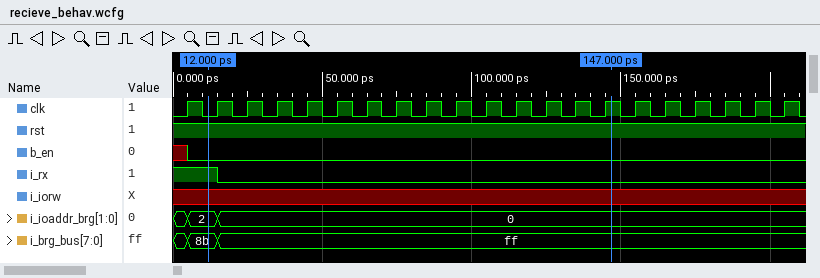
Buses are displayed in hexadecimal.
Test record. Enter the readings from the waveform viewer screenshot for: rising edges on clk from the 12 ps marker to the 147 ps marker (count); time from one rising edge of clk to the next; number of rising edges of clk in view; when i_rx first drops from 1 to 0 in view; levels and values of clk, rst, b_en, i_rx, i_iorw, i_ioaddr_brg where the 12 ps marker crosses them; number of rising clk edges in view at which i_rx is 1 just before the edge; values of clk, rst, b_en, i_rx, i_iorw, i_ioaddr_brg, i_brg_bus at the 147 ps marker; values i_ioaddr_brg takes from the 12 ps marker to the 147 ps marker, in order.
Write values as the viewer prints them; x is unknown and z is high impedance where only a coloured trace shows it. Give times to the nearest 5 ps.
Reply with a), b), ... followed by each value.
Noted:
a) 14
b) 10 ps
c) 21
d) 15 ps
e) clk=0, rst=1, b_en=0, i_rx=1, i_iorw=x, i_ioaddr_brg=2
f) 2
g) clk=1, rst=1, b_en=0, i_rx=0, i_iorw=x, i_ioaddr_brg=0, i_brg_bus=ff
h) 2, 0
